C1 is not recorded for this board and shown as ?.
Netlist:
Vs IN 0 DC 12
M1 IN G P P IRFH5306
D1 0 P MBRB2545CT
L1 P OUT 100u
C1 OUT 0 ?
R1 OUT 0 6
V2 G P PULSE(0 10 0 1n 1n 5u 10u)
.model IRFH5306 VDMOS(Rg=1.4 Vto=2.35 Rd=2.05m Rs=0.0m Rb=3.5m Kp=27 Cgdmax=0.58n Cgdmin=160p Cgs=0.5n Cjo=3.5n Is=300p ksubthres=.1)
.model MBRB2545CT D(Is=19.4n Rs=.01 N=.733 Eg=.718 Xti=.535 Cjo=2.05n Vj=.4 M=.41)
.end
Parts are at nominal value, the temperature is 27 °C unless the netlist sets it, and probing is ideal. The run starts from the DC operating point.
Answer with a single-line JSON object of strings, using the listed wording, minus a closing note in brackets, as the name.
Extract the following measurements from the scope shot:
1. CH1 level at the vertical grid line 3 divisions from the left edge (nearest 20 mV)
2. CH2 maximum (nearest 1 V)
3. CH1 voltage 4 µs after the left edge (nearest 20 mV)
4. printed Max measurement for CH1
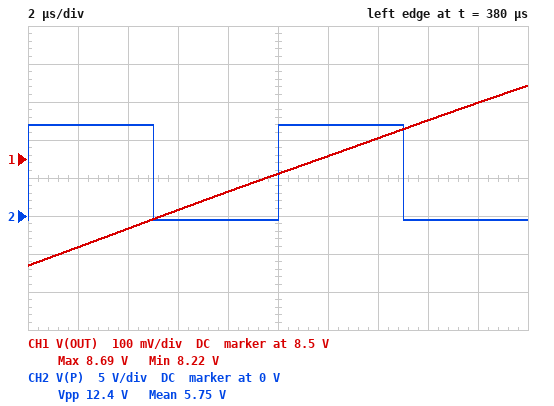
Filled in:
{"CH1 level at the vertical grid line 3 divisions from the left edge": "8.36 V", "CH2 maximum": "12 V", "CH1 voltage 4 µs after the left edge": "8.32 V", "printed Max measurement for CH1": "8.69 V"}
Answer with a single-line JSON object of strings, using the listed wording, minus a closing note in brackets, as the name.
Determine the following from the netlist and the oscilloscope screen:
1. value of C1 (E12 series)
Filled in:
{"value of C1": "330 µF"}
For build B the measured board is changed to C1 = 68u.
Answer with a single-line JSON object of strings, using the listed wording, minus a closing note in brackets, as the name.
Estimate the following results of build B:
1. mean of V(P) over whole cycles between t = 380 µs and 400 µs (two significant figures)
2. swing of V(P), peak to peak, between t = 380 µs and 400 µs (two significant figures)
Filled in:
{"mean of V(P) over whole cycles between t = 380 µs and 400 µs": "7.8 V", "swing of V(P), peak to peak, between t = 380 µs and 400 µs": "13 V"}
